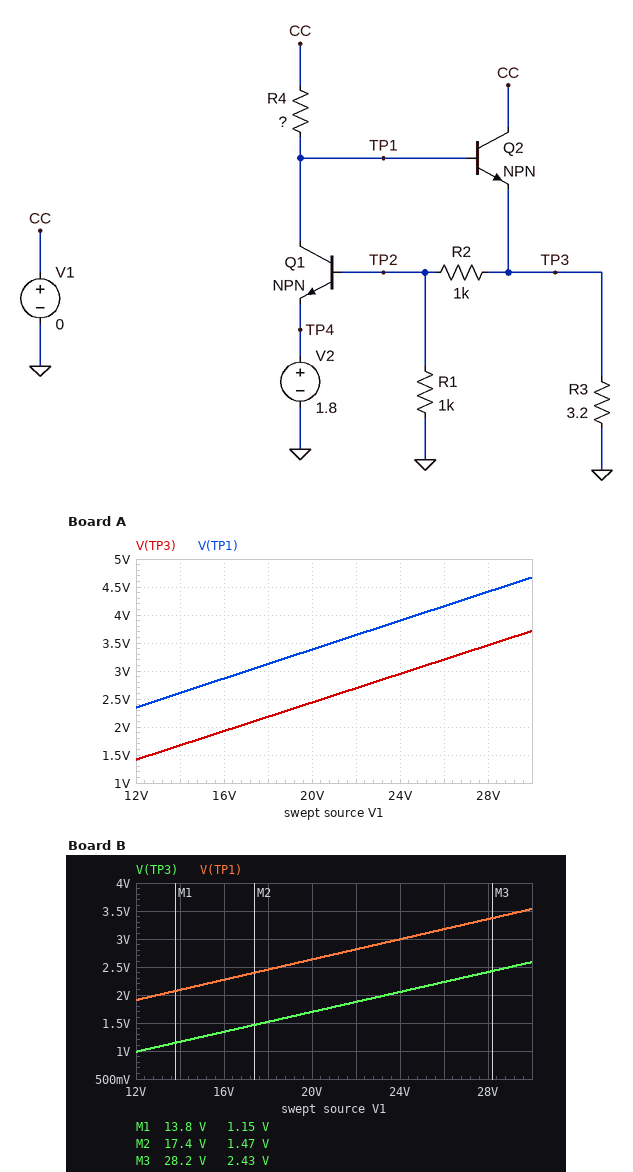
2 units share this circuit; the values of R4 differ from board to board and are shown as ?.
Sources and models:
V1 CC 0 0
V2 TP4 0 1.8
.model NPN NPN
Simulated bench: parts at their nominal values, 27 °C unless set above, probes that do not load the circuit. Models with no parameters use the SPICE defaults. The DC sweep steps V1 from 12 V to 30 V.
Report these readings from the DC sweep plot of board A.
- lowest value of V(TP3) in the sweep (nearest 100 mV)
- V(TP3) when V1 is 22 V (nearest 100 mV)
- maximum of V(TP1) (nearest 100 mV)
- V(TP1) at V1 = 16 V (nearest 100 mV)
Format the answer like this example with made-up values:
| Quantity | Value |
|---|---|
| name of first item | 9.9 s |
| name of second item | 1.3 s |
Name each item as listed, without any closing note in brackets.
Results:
| Quantity | Value |
|---|---|
| lowest value of V(TP3) in the sweep | 1.4 V |
| V(TP3) when V1 is 22 V | 2.7 V |
| maximum of V(TP1) | 4.7 V |
| V(TP1) at V1 = 16 V | 2.9 V |
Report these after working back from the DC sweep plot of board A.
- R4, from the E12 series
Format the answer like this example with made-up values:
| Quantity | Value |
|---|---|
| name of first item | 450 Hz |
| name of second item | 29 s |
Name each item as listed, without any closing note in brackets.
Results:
| Quantity | Value |
|---|---|
| R4, from the E12 series | 2.2 kΩ |
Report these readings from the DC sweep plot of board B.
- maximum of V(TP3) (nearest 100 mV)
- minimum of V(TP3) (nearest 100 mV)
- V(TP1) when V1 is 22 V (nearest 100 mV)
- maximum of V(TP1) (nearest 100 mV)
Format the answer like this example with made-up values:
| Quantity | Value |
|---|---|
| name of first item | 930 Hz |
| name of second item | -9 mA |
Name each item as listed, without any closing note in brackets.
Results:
| Quantity | Value |
|---|---|
| maximum of V(TP3) | 2.6 V |
| minimum of V(TP3) | 1.0 V |
| V(TP1) when V1 is 22 V | 2.8 V |
| maximum of V(TP1) | 3.5 V |
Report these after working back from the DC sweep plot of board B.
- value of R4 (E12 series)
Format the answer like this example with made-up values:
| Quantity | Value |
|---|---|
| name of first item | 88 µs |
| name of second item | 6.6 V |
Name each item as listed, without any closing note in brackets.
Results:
| Quantity | Value |
|---|---|
| value of R4 | 3.3 kΩ |
